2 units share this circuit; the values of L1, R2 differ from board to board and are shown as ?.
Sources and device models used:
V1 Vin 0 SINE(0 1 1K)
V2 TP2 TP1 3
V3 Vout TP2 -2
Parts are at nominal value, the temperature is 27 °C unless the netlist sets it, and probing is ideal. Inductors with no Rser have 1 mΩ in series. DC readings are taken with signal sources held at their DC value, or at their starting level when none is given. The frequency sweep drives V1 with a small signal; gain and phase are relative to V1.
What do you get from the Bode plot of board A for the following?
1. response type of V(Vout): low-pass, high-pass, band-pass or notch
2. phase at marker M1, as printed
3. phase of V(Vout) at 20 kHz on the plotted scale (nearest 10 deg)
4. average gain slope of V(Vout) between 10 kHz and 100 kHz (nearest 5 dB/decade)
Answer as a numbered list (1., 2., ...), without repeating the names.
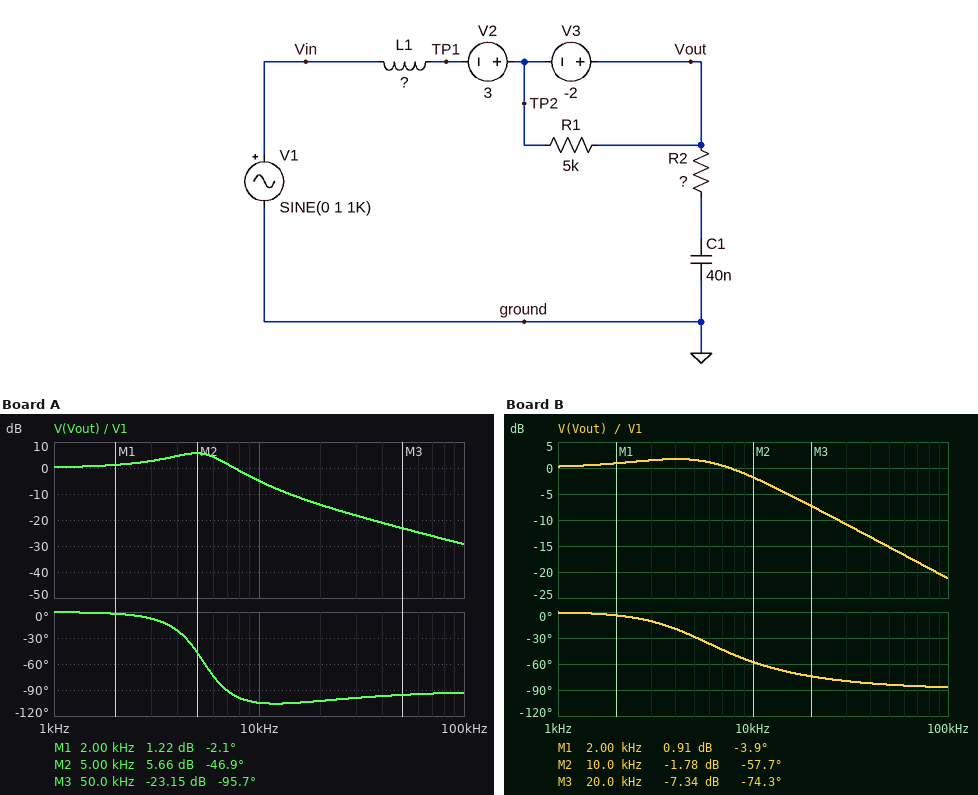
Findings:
1. low-pass
2. -2.1 deg
3. -100 deg
4. -25 dB/decade
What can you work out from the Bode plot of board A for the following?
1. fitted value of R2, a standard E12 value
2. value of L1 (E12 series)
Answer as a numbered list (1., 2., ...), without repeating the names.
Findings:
1. 470 Ω
2. 22 mH
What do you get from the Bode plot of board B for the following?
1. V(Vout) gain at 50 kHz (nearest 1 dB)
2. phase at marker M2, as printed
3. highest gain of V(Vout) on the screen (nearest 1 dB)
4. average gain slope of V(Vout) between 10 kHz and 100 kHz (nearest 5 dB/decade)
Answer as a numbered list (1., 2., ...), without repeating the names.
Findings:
1. -15 dB
2. -57.7 deg
3. 2 dB
4. -20 dB/decade
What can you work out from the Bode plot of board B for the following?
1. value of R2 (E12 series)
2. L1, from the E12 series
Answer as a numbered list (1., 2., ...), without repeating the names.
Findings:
1. 1.2 kΩ
2. 22 mH
